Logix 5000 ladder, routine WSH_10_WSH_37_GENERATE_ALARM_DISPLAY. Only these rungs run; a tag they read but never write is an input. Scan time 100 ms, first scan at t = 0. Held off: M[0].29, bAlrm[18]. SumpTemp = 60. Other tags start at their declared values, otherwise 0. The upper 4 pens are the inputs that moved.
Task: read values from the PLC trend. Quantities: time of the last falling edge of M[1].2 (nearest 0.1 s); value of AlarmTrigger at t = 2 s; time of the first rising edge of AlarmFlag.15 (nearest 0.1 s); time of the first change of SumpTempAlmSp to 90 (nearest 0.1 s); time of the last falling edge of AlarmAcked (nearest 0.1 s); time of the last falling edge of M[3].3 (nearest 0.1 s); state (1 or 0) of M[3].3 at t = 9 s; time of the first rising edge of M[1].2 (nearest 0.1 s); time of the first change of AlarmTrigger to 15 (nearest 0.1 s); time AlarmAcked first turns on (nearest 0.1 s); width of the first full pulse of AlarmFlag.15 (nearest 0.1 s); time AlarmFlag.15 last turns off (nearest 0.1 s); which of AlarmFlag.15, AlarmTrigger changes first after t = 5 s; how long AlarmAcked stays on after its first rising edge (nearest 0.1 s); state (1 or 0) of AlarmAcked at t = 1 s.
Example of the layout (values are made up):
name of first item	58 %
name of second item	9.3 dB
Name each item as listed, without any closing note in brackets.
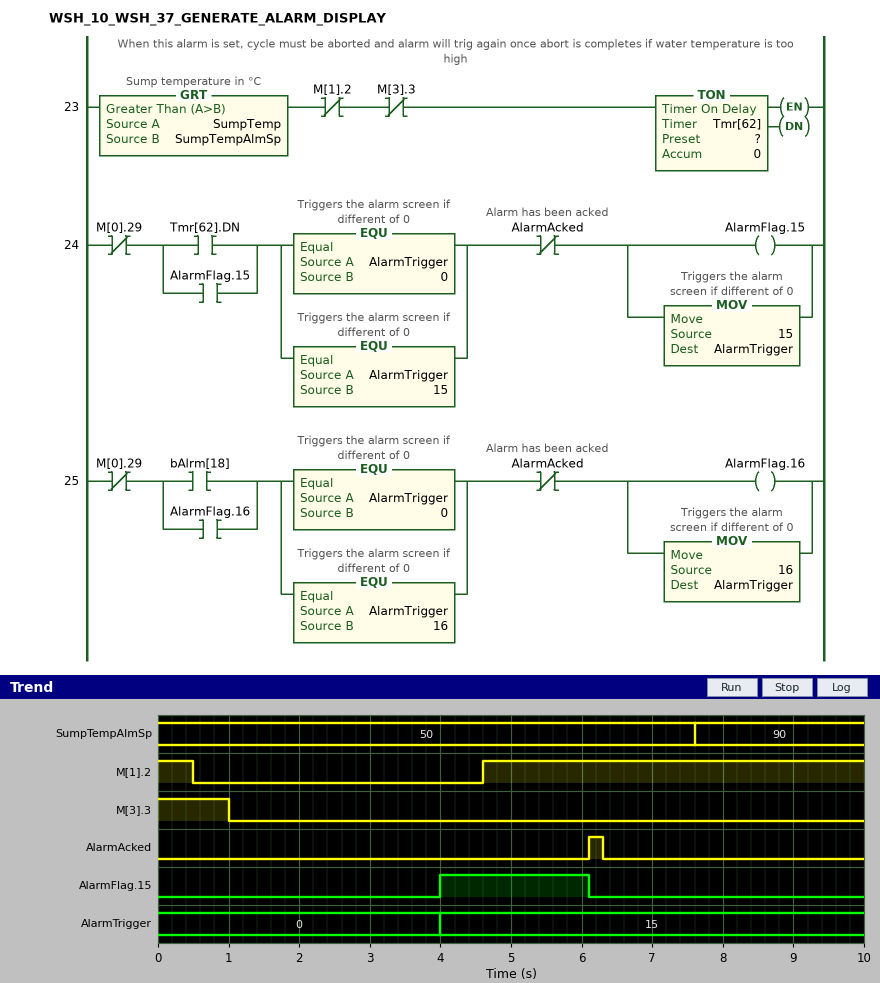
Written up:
time of the last falling edge of M[1].2	0.5 s
value of AlarmTrigger at t = 2 s	0
time of the first rising edge of AlarmFlag.15	4.0 s
time of the first change of SumpTempAlmSp to 90	7.6 s
time of the last falling edge of AlarmAcked	6.3 s
time of the last falling edge of M[3].3	1.0 s
state (1 or 0) of M[3].3 at t = 9 s	0
time of the first rising edge of M[1].2	4.6 s
time of the first change of AlarmTrigger to 15	4.0 s
time AlarmAcked first turns on	6.1 s
width of the first full pulse of AlarmFlag.15	2.1 s
time AlarmFlag.15 last turns off	6.1 s
which of AlarmFlag.15, AlarmTrigger changes first after t = 5 s	AlarmFlag.15
how long AlarmAcked stays on after its first rising edge	0.2 s
state (1 or 0) of AlarmAcked at t = 1 s	0
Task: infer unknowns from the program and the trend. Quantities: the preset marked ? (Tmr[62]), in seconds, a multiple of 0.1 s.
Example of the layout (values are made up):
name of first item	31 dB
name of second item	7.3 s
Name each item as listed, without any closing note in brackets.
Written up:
the preset marked ? (Tmr[62]), in seconds, a multiple of 0.1 s	3.0 s
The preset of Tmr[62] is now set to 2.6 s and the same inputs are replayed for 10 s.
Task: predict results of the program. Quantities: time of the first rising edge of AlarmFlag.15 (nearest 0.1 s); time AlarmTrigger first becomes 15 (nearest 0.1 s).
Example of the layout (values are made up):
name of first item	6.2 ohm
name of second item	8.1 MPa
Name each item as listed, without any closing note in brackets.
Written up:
time of the first rising edge of AlarmFlag.15	3.6 s
time AlarmTrigger first becomes 15	3.6 s
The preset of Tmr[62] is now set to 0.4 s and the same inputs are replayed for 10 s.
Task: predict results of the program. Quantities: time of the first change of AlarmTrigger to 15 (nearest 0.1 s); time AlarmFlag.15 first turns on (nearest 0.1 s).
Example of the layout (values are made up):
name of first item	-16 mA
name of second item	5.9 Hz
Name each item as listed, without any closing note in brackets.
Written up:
time of the first change of AlarmTrigger to 15	1.4 s
time AlarmFlag.15 first turns on	1.4 s
